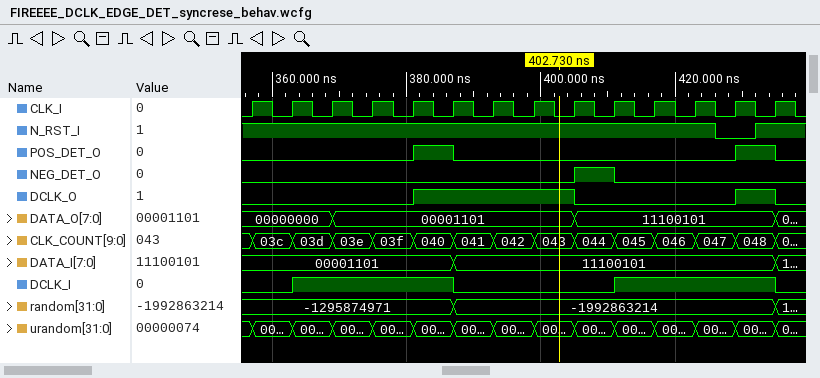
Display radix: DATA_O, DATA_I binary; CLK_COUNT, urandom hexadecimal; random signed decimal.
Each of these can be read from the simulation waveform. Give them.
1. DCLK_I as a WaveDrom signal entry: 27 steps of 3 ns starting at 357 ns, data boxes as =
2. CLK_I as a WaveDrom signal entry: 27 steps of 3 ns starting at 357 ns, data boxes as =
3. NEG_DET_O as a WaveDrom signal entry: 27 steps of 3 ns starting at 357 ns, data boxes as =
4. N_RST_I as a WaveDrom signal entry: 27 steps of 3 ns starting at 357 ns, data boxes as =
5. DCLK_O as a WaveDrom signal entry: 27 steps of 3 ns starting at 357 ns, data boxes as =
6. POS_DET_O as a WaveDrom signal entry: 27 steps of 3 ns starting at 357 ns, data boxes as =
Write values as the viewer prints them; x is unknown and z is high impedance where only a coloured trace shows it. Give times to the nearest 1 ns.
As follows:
{name: 'DCLK_I', wave: '0.1.......0.......1.......0'}
{name: 'CLK_I', wave: '101010101010101010101010101'}
{name: 'NEG_DET_O', wave: '0...............1.0........'}
{name: 'N_RST_I', wave: '1......................0.1.'}
{name: 'DCLK_O', wave: '0.......1.......0.......1.0'}
{name: 'POS_DET_O', wave: '0.......1.0.............1.0'}
